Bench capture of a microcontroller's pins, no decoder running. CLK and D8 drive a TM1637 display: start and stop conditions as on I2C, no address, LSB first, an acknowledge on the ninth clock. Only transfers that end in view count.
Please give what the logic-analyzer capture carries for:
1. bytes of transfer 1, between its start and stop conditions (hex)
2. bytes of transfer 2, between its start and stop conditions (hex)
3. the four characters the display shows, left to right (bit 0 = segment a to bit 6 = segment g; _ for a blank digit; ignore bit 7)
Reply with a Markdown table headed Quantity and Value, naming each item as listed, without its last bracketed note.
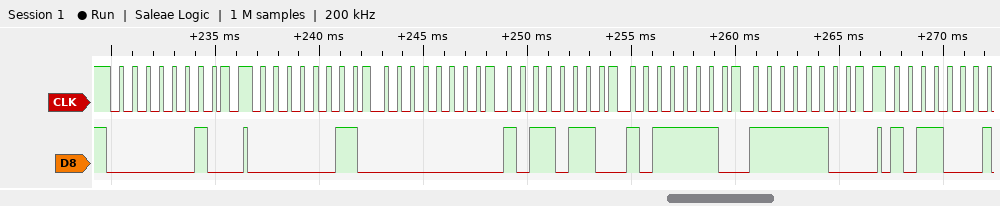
| Quantity | Value |
|---|---|
| bytes of transfer 1, between its start and stop conditions | 40 |
| bytes of transfer 2, between its start and stop conditions | C0 00 6D 7D 3F |
| the four characters the display shows, left to right | _560 |
